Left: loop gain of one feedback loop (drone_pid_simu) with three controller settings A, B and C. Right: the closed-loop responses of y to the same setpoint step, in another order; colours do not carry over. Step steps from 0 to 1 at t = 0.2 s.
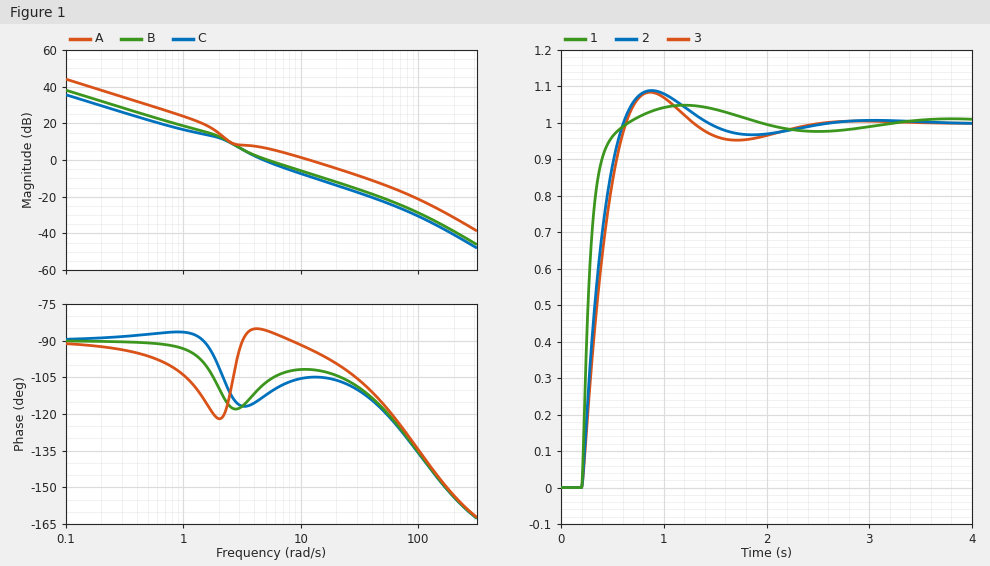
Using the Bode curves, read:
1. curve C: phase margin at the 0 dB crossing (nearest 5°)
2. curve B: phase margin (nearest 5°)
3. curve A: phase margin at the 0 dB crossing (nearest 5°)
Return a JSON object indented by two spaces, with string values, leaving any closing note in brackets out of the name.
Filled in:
{
  "curve C: phase margin at the 0 dB crossing": "65°",
  "curve B: phase margin": "75°",
  "curve A: phase margin at the 0 dB crossing": "85°"
}
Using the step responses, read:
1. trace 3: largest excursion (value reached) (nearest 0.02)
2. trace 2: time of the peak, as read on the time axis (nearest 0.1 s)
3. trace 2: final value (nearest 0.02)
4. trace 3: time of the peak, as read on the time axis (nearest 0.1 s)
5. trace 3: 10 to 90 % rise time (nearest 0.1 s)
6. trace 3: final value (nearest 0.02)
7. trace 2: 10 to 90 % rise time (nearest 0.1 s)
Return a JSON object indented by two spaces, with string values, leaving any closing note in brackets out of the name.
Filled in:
{
  "trace 3: largest excursion (value reached)": "1.08",
  "trace 2: time of the peak, as read on the time axis": "0.9 s",
  "trace 2: final value": "1.00",
  "trace 3: time of the peak, as read on the time axis": "0.9 s",
  "trace 3: 10 to 90 % rise time": "0.3 s",
  "trace 3: final value": "1.00",
  "trace 2: 10 to 90 % rise time": "0.3 s"
}
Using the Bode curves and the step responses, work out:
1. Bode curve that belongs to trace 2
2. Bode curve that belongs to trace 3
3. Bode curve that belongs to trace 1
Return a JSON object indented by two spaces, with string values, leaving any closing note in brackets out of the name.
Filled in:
{
  "Bode curve that belongs to trace 2": "B",
  "Bode curve that belongs to trace 3": "C",
  "Bode curve that belongs to trace 1": "A"
}
